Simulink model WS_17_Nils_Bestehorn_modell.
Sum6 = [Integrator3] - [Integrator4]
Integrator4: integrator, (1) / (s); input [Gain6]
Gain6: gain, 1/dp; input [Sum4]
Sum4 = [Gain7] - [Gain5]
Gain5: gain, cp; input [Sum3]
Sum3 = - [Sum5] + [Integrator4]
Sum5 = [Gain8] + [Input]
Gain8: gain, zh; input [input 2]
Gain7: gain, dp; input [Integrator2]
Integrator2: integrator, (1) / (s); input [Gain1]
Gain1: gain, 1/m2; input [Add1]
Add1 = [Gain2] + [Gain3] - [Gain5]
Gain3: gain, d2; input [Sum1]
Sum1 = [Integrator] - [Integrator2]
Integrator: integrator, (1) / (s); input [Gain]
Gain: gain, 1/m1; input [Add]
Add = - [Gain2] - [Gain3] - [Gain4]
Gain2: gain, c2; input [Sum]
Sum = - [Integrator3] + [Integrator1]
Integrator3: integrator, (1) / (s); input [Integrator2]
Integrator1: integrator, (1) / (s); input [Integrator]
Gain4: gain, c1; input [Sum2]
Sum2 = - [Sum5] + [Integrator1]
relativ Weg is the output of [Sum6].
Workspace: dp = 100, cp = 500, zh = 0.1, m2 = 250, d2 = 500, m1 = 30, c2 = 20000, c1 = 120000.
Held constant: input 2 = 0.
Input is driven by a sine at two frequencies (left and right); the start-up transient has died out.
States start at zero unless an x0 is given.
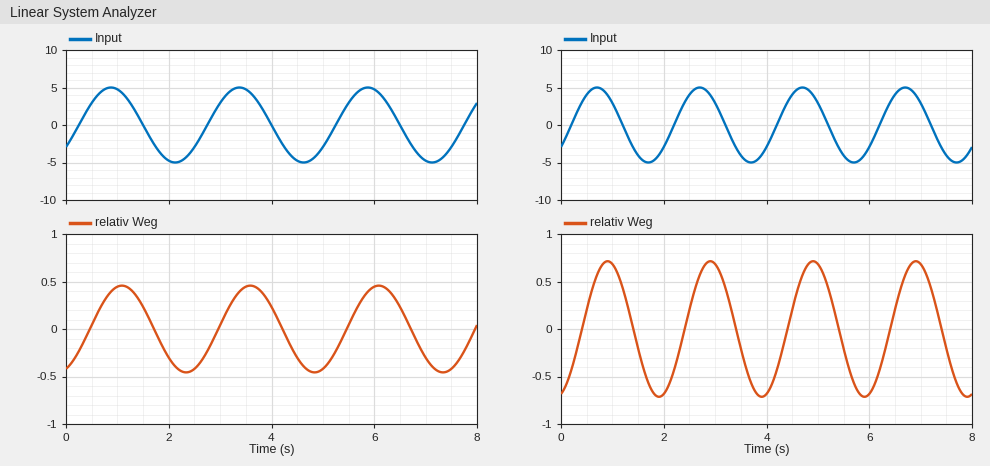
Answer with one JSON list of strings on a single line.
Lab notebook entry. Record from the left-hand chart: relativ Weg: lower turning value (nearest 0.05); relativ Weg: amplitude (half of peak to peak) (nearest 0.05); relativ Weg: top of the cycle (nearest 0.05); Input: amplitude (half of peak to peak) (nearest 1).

["-0.45", "0.45", "0.45", "5"]
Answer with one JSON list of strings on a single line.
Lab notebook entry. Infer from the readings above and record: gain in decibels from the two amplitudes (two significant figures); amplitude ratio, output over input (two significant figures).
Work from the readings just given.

["-21 dB", "0.090"]
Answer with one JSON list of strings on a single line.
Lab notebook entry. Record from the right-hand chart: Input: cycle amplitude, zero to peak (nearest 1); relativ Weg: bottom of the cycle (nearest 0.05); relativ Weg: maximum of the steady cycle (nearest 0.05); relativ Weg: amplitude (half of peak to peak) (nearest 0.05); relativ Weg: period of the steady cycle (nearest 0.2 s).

["5", "-0.70", "0.70", "0.70", "2.0 s"]
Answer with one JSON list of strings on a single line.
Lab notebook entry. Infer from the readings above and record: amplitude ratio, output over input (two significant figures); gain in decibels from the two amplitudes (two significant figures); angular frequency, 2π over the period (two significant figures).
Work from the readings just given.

["0.14", "-17 dB", "3.1 rad/s"]
